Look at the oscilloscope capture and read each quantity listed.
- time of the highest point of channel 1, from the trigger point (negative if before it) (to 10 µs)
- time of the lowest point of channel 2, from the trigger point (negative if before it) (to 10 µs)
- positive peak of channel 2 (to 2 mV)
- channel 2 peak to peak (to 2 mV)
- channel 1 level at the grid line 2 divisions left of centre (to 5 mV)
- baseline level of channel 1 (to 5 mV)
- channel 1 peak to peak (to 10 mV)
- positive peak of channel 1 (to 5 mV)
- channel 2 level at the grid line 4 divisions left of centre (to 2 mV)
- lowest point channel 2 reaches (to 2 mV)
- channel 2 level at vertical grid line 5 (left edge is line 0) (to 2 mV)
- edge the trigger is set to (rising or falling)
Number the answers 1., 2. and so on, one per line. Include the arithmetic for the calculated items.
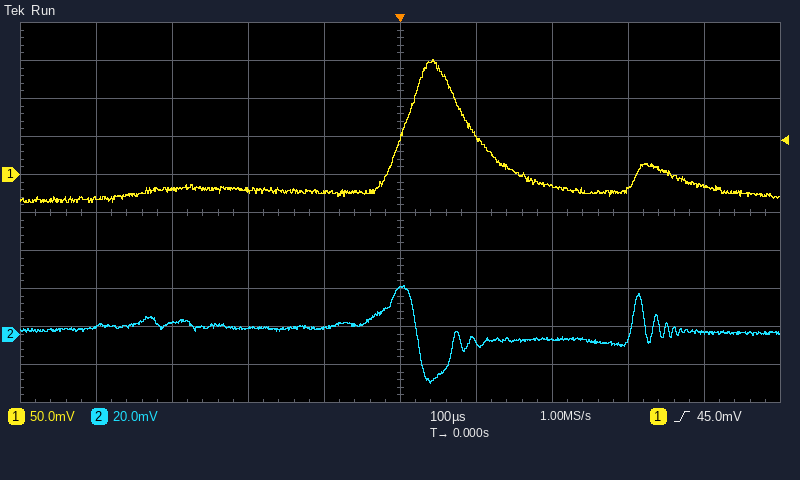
1. +40 µs
2. +40 µs
3. 26 mV
4. 26 mV − (-26 mV) = 52 mV
5. -20 mV
6. -20 mV
7. 190 mV
8. 150 mV
9. 4 mV
10. -26 mV
11. 24 mV
12. rising
